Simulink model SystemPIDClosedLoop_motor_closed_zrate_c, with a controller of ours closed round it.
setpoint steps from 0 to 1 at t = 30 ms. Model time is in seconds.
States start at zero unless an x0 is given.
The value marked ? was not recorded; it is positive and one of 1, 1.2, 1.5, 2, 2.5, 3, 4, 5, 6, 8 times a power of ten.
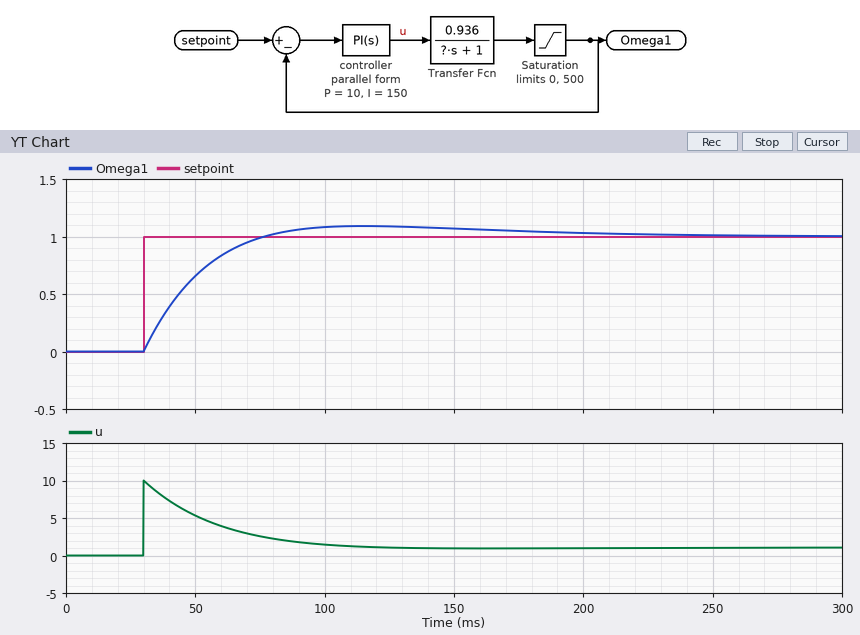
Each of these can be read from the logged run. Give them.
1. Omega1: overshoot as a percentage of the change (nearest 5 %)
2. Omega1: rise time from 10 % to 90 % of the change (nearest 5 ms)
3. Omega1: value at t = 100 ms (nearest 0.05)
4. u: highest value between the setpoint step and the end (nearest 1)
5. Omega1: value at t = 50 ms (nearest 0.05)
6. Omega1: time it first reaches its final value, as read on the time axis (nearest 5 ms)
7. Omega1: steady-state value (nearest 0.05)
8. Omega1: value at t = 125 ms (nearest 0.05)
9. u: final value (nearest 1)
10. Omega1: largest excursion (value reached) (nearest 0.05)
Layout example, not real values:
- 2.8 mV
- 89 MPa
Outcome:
- 10 %
- 35 ms
- 1.10
- 10
- 0.65
- 75 ms
- 1.00
- 1.10
- 1
- 1.10
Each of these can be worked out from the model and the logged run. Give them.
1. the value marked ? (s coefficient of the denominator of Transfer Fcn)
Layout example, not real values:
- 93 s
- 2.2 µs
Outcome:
- 0.2
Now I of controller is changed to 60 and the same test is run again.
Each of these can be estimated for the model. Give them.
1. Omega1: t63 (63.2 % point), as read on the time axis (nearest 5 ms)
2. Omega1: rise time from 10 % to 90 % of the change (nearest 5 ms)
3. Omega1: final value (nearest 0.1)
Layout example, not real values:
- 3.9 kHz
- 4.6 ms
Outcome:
- 50 ms
- 45 ms
- 1.0
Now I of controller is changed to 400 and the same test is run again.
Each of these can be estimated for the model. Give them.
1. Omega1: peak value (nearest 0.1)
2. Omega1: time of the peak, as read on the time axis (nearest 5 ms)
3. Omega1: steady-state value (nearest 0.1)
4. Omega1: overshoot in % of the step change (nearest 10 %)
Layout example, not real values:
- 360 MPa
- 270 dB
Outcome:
- 1.2
- 85 ms
- 1.0
- 20 %
